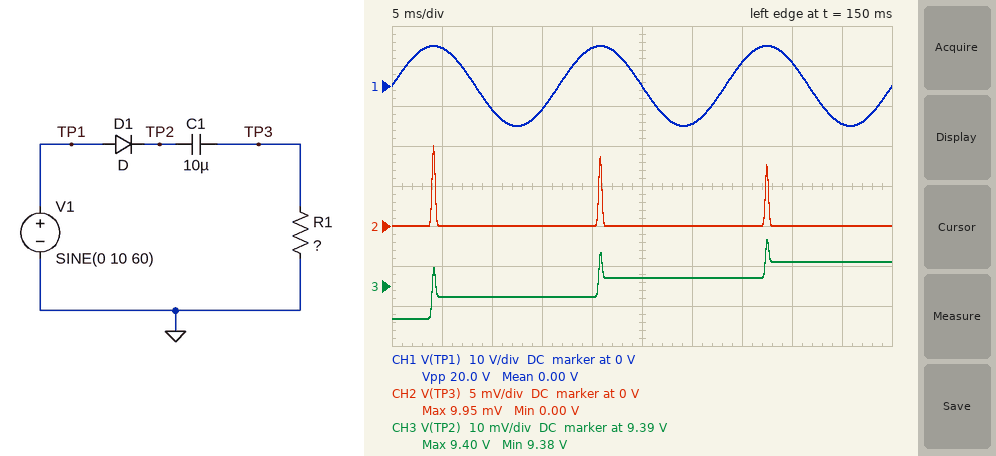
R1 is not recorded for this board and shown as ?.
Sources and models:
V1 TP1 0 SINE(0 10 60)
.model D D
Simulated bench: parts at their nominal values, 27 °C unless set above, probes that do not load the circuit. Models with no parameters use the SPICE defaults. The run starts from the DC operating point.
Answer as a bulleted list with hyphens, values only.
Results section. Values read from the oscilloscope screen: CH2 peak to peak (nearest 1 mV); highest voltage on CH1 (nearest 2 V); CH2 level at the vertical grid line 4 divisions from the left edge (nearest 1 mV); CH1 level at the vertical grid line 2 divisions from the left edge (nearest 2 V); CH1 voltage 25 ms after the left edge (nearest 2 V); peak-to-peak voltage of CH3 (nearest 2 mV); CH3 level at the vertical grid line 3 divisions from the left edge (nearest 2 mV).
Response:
- 10 mV
- 10 V
- 0 V
- -6 V
- 0 V
- 20 mV
- 9.388 V
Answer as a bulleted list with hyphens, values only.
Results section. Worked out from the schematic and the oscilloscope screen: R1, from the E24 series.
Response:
- 68 Ω
